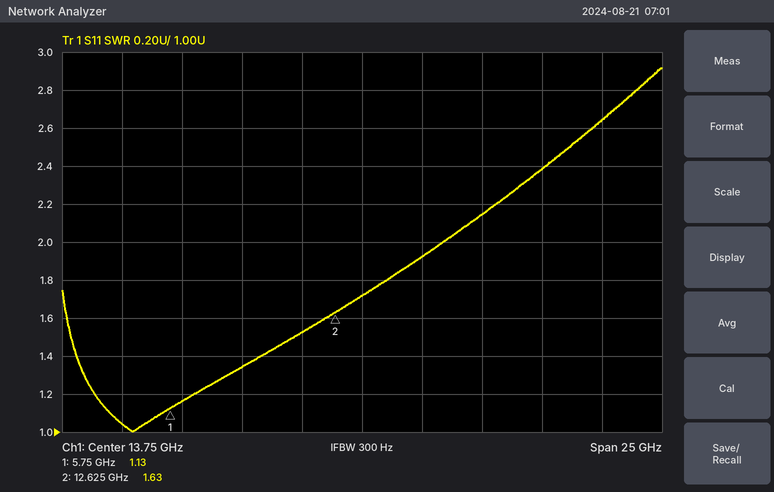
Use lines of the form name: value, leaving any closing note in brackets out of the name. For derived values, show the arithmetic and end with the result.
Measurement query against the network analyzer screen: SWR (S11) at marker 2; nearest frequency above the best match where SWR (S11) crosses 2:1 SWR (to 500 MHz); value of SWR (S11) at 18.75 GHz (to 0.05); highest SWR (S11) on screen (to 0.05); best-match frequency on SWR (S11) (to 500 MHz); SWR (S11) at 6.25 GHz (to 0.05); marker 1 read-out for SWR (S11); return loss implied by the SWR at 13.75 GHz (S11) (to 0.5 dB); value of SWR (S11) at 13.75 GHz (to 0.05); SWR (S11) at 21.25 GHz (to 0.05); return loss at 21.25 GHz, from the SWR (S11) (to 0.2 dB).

SWR (S11) at marker 2: 1.63
nearest frequency above the best match where SWR (S11) crosses 2:1 SWR: 17.0 GHz
value of SWR (S11) at 18.75 GHz: 2.15
highest SWR (S11) on screen: 2.90
best-match frequency on SWR (S11): 4.0 GHz
SWR (S11) at 6.25 GHz: 1.15
marker 1 read-out for SWR: 1.13
return loss implied by the SWR at 13.75 GHz (S11): −20 log10((1.7 − 1)/(1.7 + 1)) ≈ 11.7 dB, so 11.5 dB to the nearest 0.5 dB
value of SWR (S11) at 13.75 GHz: 1.70
SWR (S11) at 21.25 GHz: 2.40
return loss at 21.25 GHz, from the SWR (S11): −20 log10((2.4 − 1)/(2.4 + 1)) ≈ 7.71 dB, so 7.8 dB to the nearest 0.2 dB
